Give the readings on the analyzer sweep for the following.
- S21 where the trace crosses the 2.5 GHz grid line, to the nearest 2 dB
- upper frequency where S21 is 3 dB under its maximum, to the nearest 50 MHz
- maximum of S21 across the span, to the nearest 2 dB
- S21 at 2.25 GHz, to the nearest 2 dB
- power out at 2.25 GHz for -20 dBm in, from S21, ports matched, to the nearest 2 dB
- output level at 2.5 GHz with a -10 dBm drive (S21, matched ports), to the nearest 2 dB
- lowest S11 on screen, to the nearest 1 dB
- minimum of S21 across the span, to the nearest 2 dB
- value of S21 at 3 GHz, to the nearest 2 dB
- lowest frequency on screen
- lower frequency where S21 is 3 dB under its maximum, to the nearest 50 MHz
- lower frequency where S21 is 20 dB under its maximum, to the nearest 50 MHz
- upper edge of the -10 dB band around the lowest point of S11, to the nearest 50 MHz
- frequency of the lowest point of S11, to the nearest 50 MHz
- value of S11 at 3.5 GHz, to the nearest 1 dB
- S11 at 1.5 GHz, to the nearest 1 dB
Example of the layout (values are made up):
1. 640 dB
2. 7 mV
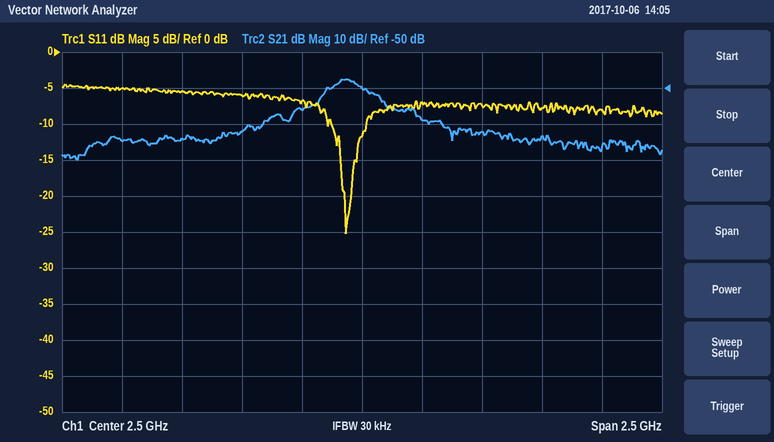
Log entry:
1. -50 dB
2. 2.50 GHz
3. -48 dB
4. -56 dB
5. -76 dBm
6. -60 dBm
7. -25 dB
8. -70 dB
9. -62 dB
10. 1.25 GHz
11. 2.35 GHz
12. 1.35 GHz
13. 2.50 GHz
14. 2.45 GHz
15. -8 dB
16. -5 dB
